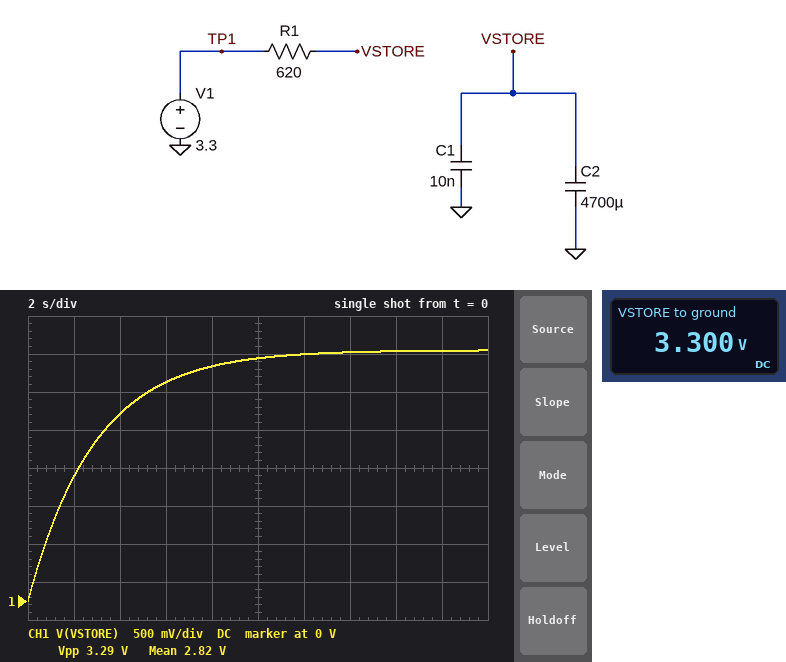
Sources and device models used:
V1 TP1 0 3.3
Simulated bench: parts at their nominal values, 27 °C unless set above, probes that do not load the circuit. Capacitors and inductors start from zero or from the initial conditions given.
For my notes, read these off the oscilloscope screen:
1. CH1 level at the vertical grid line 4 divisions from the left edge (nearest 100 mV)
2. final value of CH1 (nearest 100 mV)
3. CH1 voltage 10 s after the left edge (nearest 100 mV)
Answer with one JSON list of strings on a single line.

["3.1 V", "3.3 V", "3.2 V"]
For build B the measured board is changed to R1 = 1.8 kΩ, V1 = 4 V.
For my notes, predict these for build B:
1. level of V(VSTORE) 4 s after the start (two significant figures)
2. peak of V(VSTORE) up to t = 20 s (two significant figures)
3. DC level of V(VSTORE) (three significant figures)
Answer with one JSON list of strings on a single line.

["1.5 V", "3.6 V", "4.00 V"]
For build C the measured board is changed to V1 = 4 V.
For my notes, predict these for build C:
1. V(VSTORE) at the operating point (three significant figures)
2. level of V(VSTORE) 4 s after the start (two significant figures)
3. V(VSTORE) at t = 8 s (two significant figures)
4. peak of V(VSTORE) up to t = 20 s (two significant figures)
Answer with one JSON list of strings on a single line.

["4.00 V", "3.0 V", "3.7 V", "4.0 V"]
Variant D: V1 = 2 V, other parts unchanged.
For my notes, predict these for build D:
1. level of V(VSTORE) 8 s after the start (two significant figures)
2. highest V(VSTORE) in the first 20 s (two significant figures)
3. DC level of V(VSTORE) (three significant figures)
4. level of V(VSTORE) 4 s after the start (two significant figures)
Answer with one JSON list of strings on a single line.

["1.9 V", "2.0 V", "2.00 V", "1.5 V"]
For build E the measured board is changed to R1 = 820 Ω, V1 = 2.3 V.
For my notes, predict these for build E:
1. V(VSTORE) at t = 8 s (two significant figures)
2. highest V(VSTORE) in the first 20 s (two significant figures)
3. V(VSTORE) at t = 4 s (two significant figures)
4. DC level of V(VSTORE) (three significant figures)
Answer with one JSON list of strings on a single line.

["2.0 V", "2.3 V", "1.5 V", "2.30 V"]
